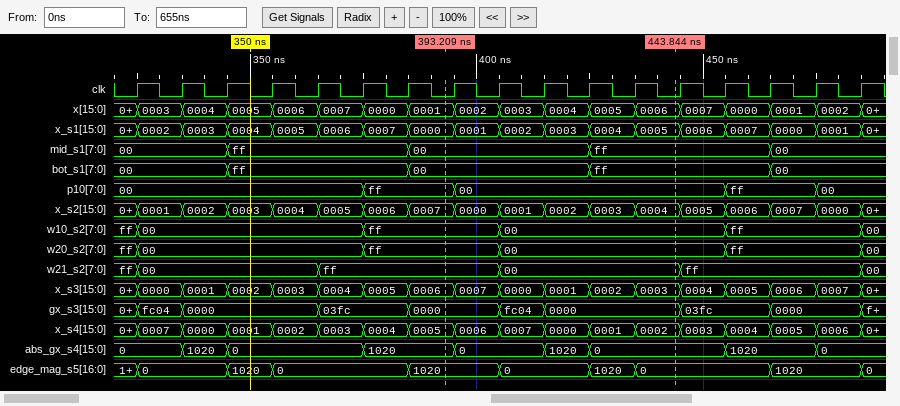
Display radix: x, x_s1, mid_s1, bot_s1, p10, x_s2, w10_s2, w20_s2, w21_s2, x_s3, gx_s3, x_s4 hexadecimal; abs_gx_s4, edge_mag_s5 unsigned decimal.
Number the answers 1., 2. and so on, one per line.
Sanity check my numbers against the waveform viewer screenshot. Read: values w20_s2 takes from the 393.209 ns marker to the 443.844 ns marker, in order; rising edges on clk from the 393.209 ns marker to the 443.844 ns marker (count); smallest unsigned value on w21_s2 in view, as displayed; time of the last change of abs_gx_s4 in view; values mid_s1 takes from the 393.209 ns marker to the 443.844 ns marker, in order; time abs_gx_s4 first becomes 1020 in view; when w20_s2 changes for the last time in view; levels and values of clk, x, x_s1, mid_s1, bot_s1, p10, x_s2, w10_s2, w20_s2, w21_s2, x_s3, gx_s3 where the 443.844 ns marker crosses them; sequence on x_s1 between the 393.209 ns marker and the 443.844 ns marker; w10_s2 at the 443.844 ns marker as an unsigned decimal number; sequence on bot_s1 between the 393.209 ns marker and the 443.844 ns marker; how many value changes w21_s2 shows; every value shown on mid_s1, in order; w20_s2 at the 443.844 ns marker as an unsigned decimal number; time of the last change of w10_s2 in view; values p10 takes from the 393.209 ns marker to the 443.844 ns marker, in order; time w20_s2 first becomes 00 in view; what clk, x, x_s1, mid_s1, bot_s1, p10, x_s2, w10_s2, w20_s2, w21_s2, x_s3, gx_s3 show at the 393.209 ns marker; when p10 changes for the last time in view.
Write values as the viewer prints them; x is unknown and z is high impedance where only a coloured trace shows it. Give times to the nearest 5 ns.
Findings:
1. ff, 00
2. 5
3. 00
4. 475 ns
5. 00, ff
6. 335 ns
7. 485 ns
8. clk=0, x=0006, x_s1=0005, mid_s1=ff, bot_s1=ff, p10=00, x_s2=0004, w10_s2=00, w20_s2=00, w21_s2=00, x_s3=0003, gx_s3=0000
9. 0000, 0001, 0002, 0003, 0004, 0005
10. 0
11. 00, ff
12. 5
13. 00, ff, 00, ff, 00
14. 0
15. 485 ns
16. ff, 00
17. 325 ns
18. clk=0, x=0001, x_s1=0000, mid_s1=00, bot_s1=00, p10=ff, x_s2=0007, w10_s2=ff, w20_s2=ff, w21_s2=ff, x_s3=0006, gx_s3=0000
19. 475 ns
